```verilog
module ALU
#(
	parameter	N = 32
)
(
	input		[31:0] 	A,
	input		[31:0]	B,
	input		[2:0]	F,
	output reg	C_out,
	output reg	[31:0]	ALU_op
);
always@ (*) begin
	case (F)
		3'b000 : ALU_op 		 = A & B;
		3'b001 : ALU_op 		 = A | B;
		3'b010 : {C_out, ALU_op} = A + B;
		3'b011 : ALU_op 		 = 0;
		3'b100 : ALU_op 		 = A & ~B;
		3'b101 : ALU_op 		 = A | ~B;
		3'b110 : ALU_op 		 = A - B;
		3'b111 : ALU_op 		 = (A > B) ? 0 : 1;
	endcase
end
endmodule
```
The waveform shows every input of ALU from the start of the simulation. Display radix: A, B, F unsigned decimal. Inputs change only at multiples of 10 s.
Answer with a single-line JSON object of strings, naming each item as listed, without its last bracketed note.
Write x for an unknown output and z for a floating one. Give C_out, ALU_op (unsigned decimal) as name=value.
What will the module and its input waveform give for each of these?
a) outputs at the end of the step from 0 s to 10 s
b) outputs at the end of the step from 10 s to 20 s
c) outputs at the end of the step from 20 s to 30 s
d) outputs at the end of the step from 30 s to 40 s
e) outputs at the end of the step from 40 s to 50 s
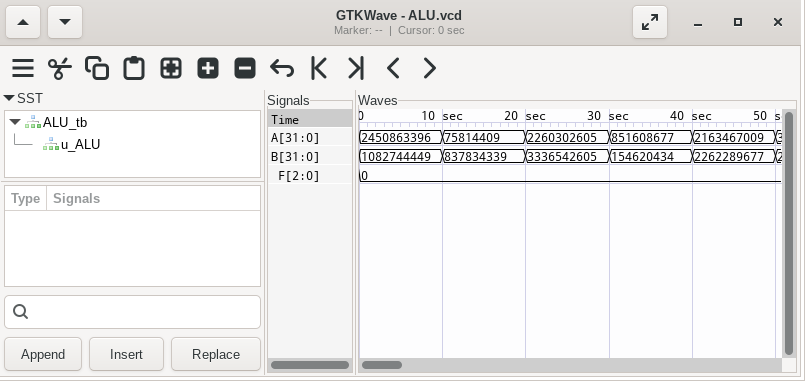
{"outputs at the end of the step from 0 s to 10 s": "C_out=x, ALU_op=70656", "outputs at the end of the step from 10 s to 20 s": "C_out=x, ALU_op=8410625", "outputs at the end of the step from 20 s to 30 s": "C_out=x, ALU_op=2258180365", "outputs at the end of the step from 30 s to 40 s": "C_out=x, ALU_op=131072", "outputs at the end of the step from 40 s to 50 s": "C_out=x, ALU_op=2161361153"}
